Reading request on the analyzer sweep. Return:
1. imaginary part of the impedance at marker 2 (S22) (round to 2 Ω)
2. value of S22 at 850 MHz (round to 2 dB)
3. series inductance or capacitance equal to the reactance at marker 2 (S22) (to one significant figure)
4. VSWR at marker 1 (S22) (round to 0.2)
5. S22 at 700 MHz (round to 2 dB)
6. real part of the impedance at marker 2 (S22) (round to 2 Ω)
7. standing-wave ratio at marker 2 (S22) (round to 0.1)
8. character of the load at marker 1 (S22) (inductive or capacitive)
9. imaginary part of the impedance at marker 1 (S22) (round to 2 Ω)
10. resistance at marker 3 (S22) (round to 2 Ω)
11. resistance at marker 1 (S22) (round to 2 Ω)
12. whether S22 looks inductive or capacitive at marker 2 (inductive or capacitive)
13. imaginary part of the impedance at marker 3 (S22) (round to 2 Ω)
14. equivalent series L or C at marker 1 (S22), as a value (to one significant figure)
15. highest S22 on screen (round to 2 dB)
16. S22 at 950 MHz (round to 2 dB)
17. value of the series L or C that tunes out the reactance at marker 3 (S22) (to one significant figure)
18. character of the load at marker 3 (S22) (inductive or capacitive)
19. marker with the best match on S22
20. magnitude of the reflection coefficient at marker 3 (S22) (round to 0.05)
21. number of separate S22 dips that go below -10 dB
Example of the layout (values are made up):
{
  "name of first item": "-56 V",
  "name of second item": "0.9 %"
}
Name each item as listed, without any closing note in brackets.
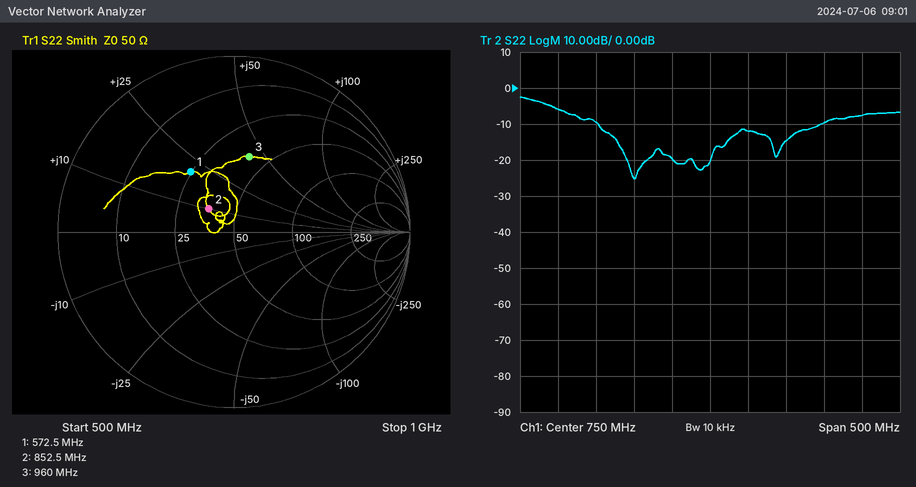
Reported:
{
  "imaginary part of the impedance at marker 2 (S22)": "+10 Ω",
  "value of S22 at 850 MHz": "-14 dB",
  "series inductance or capacitance equal to the reactance at marker 2 (S22)": "2 nH",
  "VSWR at marker 1 (S22)": "2.4",
  "S22 at 700 MHz": "-20 dB",
  "real part of the impedance at marker 2 (S22)": "36 Ω",
  "standing-wave ratio at marker 2 (S22)": "1.5",
  "character of the load at marker 1 (S22)": "inductive",
  "imaginary part of the impedance at marker 1 (S22)": "+20 Ω",
  "resistance at marker 3 (S22)": "40 Ω",
  "resistance at marker 1 (S22)": "24 Ω",
  "whether S22 looks inductive or capacitive at marker 2": "inductive",
  "imaginary part of the impedance at marker 3 (S22)": "+42 Ω",
  "equivalent series L or C at marker 1 (S22), as a value": "6 nH",
  "highest S22 on screen": "-2 dB",
  "S22 at 950 MHz": "-8 dB",
  "value of the series L or C that tunes out the reactance at marker 3 (S22)": "4 pF",
  "character of the load at marker 3 (S22)": "inductive",
  "marker with the best match on S22": "marker 2",
  "magnitude of the reflection coefficient at marker 3 (S22)": "0.45",
  "number of separate S22 dips that go below -10 dB": "3"
}
